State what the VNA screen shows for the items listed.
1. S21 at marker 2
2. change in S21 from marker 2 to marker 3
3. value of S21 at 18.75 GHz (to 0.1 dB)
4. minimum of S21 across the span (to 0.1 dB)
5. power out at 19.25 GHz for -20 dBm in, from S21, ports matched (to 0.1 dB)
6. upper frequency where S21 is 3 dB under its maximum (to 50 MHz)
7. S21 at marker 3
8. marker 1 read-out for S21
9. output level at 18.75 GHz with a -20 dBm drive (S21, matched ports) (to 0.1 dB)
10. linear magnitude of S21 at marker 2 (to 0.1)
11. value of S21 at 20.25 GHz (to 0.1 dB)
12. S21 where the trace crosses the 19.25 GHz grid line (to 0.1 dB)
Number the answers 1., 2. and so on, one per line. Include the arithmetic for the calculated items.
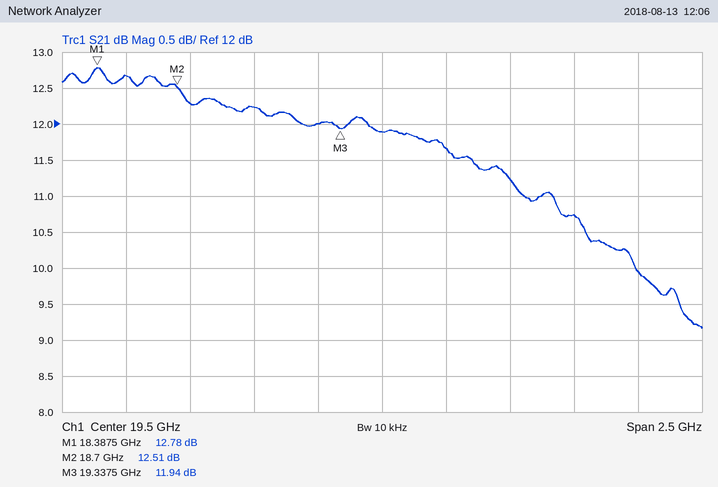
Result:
1. 12.51 dB
2. 11.94 − (12.51) = -0.57 dB
3. 12.3 dB
4. 9.2 dB
5. -20 dBm + (12.0 dB) = -8.0 dBm
6. 20.55 GHz
7. 11.94 dB
8. 12.78 dB
9. -20 dBm + (12.3 dB) = -7.7 dBm
10. 10^(12.51/20) ≈ 4.2
11. 10.7 dB
12. 12.0 dB
